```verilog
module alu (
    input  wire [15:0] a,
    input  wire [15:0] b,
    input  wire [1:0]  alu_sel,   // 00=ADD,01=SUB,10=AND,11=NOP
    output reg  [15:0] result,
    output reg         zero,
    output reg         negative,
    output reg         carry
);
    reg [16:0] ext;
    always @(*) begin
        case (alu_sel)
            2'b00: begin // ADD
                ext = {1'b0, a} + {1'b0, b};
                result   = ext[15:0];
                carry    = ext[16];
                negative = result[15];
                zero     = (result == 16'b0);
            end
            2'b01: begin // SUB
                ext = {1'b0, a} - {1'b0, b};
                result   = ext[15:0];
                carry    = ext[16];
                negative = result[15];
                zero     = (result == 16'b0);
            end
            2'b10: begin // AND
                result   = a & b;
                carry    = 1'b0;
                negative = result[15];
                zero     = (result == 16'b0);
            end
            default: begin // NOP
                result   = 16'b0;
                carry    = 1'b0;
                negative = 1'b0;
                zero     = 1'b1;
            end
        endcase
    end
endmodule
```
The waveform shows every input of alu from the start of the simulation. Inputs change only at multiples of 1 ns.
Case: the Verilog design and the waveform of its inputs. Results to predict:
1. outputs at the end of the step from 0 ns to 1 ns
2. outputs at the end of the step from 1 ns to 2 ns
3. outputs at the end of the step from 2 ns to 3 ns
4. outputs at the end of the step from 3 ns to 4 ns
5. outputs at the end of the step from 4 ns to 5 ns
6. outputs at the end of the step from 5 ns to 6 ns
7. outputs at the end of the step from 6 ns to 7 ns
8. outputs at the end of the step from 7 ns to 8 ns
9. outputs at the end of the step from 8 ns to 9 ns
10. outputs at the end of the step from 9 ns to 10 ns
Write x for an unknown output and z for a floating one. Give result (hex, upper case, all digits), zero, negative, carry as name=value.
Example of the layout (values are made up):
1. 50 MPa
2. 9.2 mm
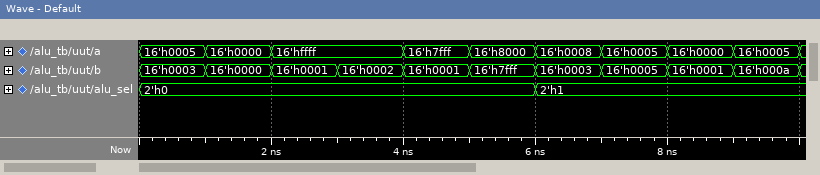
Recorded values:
1. result=0008, zero=0, negative=0, carry=0
2. result=0000, zero=1, negative=0, carry=0
3. result=0000, zero=1, negative=0, carry=1
4. result=0001, zero=0, negative=0, carry=1
5. result=8000, zero=0, negative=1, carry=0
6. result=FFFF, zero=0, negative=1, carry=0
7. result=0005, zero=0, negative=0, carry=0
8. result=0000, zero=1, negative=0, carry=0
9. result=FFFF, zero=0, negative=1, carry=1
10. result=FFFB, zero=0, negative=1, carry=1
